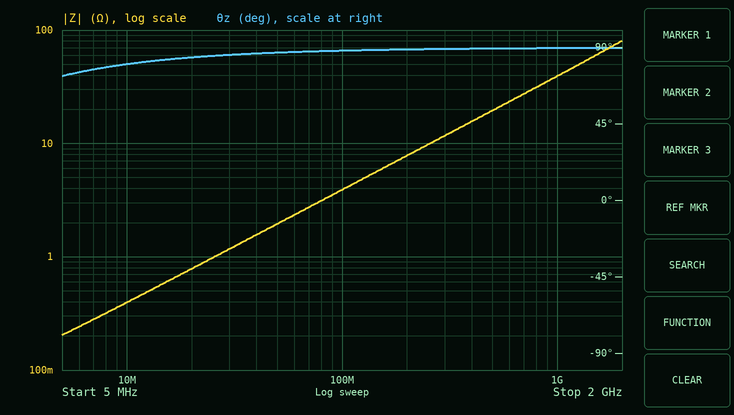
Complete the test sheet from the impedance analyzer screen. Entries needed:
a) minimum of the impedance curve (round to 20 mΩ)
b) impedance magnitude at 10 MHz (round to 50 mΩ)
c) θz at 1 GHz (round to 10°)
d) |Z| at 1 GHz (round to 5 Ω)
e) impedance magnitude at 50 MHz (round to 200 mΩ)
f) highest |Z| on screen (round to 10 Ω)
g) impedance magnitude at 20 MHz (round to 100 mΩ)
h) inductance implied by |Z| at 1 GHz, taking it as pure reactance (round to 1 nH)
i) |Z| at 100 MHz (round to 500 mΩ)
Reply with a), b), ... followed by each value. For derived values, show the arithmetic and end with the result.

a) 200 mΩ
b) 400 mΩ
c) 90°
d) 40 Ω
e) 2.0 Ω
f) 80 Ω
g) 800 mΩ
h) L = 40 Ω/(2π × 1 GHz) ≈ 6 nH
i) 4.0 Ω
